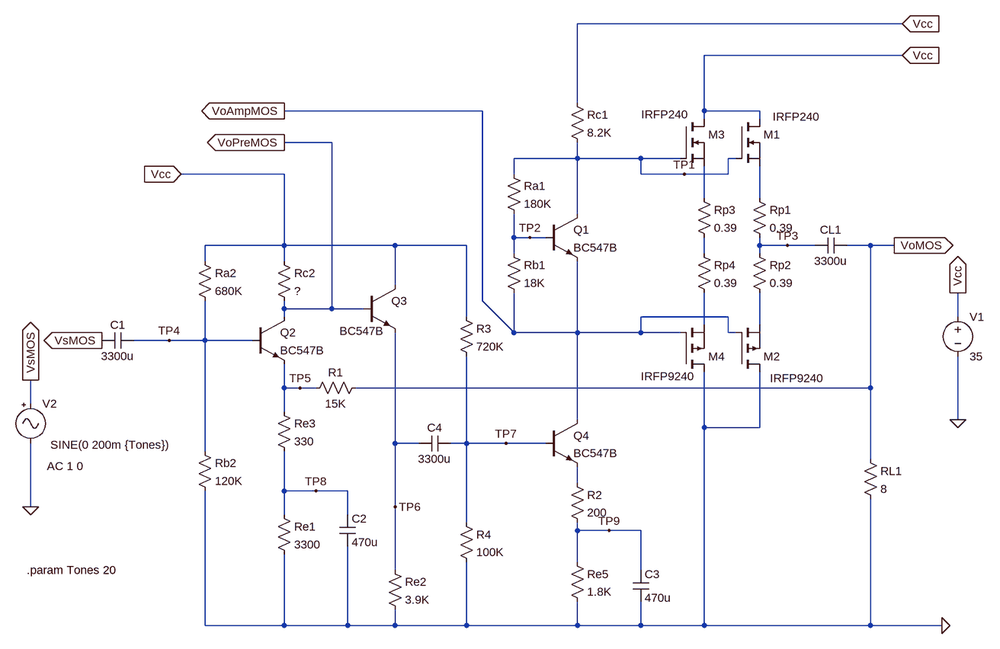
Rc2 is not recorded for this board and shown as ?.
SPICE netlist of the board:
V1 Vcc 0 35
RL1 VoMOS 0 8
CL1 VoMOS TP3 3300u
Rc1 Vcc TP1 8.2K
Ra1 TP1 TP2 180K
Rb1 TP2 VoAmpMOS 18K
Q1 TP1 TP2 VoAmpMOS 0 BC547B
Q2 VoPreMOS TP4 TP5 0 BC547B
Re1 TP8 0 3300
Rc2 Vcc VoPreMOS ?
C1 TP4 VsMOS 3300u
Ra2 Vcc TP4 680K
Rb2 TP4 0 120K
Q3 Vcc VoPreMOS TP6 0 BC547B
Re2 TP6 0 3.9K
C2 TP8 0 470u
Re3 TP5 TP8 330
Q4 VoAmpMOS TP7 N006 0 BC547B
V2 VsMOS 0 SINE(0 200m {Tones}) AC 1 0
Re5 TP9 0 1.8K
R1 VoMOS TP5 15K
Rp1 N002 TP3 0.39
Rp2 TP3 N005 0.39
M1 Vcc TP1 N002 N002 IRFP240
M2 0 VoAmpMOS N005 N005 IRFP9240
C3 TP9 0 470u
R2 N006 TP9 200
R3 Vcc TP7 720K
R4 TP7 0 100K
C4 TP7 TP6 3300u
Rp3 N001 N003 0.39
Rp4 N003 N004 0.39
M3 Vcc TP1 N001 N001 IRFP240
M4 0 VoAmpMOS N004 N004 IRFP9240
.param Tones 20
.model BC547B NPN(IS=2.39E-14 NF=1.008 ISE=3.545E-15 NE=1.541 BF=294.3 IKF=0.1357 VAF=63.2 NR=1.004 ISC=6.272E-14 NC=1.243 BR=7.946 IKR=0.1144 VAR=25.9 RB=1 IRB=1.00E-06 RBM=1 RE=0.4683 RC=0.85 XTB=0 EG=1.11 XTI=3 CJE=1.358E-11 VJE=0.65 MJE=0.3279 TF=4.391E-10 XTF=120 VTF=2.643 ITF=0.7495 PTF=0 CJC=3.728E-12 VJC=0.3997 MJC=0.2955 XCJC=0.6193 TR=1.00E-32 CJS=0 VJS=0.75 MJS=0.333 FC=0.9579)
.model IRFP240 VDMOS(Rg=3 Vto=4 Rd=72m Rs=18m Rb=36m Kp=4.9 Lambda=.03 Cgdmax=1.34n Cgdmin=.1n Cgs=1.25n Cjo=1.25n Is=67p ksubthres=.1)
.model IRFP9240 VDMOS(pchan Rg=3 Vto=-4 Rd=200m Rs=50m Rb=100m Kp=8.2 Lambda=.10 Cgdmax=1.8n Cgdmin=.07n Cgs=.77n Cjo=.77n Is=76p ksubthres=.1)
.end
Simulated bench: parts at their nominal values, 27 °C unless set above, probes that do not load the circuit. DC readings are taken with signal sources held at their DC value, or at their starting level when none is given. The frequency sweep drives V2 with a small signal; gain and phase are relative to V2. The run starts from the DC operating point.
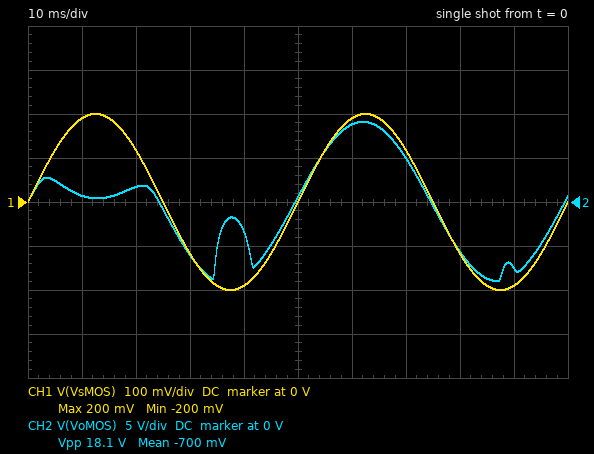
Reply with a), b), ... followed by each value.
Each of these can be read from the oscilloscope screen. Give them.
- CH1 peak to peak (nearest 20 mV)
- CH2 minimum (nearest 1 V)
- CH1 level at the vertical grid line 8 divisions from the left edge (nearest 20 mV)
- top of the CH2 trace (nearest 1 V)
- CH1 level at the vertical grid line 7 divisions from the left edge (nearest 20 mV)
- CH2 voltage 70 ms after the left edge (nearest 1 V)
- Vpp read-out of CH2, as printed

a) 400 mV
b) -9 V
c) -120 mV
d) 9 V
e) 120 mV
f) 5 V
g) 18.1 V
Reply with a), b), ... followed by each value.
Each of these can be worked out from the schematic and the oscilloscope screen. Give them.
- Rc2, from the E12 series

a) 22 kΩ
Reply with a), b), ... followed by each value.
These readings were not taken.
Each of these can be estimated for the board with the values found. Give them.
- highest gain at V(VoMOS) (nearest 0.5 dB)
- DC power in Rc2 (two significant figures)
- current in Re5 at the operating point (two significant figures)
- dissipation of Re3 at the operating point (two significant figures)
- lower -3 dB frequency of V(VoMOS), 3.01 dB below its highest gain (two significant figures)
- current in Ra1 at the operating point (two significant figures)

a) 37.5 dB
b) 43 mW
c) 1.6 mA
d) 420 µW
e) 340 kHz
f) 41 µA
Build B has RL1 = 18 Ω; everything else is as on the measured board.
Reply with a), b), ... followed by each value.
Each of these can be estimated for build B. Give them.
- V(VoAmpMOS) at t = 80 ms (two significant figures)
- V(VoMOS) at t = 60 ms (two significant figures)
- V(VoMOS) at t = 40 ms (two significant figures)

a) 7.2 V
b) 4.8 V
c) -8.7 V
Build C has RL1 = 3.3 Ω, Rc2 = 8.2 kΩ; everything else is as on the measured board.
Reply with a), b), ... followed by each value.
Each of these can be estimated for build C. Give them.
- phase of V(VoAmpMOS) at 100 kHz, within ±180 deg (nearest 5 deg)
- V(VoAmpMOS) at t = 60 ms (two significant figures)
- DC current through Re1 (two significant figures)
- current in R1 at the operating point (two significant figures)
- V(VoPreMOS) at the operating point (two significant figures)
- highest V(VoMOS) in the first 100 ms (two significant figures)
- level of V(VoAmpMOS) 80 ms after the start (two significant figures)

a) -15 deg
b) 25 V
c) 1.2 mA
d) 280 µA
e) 23 V
f) 8.2 V
g) 12 V
